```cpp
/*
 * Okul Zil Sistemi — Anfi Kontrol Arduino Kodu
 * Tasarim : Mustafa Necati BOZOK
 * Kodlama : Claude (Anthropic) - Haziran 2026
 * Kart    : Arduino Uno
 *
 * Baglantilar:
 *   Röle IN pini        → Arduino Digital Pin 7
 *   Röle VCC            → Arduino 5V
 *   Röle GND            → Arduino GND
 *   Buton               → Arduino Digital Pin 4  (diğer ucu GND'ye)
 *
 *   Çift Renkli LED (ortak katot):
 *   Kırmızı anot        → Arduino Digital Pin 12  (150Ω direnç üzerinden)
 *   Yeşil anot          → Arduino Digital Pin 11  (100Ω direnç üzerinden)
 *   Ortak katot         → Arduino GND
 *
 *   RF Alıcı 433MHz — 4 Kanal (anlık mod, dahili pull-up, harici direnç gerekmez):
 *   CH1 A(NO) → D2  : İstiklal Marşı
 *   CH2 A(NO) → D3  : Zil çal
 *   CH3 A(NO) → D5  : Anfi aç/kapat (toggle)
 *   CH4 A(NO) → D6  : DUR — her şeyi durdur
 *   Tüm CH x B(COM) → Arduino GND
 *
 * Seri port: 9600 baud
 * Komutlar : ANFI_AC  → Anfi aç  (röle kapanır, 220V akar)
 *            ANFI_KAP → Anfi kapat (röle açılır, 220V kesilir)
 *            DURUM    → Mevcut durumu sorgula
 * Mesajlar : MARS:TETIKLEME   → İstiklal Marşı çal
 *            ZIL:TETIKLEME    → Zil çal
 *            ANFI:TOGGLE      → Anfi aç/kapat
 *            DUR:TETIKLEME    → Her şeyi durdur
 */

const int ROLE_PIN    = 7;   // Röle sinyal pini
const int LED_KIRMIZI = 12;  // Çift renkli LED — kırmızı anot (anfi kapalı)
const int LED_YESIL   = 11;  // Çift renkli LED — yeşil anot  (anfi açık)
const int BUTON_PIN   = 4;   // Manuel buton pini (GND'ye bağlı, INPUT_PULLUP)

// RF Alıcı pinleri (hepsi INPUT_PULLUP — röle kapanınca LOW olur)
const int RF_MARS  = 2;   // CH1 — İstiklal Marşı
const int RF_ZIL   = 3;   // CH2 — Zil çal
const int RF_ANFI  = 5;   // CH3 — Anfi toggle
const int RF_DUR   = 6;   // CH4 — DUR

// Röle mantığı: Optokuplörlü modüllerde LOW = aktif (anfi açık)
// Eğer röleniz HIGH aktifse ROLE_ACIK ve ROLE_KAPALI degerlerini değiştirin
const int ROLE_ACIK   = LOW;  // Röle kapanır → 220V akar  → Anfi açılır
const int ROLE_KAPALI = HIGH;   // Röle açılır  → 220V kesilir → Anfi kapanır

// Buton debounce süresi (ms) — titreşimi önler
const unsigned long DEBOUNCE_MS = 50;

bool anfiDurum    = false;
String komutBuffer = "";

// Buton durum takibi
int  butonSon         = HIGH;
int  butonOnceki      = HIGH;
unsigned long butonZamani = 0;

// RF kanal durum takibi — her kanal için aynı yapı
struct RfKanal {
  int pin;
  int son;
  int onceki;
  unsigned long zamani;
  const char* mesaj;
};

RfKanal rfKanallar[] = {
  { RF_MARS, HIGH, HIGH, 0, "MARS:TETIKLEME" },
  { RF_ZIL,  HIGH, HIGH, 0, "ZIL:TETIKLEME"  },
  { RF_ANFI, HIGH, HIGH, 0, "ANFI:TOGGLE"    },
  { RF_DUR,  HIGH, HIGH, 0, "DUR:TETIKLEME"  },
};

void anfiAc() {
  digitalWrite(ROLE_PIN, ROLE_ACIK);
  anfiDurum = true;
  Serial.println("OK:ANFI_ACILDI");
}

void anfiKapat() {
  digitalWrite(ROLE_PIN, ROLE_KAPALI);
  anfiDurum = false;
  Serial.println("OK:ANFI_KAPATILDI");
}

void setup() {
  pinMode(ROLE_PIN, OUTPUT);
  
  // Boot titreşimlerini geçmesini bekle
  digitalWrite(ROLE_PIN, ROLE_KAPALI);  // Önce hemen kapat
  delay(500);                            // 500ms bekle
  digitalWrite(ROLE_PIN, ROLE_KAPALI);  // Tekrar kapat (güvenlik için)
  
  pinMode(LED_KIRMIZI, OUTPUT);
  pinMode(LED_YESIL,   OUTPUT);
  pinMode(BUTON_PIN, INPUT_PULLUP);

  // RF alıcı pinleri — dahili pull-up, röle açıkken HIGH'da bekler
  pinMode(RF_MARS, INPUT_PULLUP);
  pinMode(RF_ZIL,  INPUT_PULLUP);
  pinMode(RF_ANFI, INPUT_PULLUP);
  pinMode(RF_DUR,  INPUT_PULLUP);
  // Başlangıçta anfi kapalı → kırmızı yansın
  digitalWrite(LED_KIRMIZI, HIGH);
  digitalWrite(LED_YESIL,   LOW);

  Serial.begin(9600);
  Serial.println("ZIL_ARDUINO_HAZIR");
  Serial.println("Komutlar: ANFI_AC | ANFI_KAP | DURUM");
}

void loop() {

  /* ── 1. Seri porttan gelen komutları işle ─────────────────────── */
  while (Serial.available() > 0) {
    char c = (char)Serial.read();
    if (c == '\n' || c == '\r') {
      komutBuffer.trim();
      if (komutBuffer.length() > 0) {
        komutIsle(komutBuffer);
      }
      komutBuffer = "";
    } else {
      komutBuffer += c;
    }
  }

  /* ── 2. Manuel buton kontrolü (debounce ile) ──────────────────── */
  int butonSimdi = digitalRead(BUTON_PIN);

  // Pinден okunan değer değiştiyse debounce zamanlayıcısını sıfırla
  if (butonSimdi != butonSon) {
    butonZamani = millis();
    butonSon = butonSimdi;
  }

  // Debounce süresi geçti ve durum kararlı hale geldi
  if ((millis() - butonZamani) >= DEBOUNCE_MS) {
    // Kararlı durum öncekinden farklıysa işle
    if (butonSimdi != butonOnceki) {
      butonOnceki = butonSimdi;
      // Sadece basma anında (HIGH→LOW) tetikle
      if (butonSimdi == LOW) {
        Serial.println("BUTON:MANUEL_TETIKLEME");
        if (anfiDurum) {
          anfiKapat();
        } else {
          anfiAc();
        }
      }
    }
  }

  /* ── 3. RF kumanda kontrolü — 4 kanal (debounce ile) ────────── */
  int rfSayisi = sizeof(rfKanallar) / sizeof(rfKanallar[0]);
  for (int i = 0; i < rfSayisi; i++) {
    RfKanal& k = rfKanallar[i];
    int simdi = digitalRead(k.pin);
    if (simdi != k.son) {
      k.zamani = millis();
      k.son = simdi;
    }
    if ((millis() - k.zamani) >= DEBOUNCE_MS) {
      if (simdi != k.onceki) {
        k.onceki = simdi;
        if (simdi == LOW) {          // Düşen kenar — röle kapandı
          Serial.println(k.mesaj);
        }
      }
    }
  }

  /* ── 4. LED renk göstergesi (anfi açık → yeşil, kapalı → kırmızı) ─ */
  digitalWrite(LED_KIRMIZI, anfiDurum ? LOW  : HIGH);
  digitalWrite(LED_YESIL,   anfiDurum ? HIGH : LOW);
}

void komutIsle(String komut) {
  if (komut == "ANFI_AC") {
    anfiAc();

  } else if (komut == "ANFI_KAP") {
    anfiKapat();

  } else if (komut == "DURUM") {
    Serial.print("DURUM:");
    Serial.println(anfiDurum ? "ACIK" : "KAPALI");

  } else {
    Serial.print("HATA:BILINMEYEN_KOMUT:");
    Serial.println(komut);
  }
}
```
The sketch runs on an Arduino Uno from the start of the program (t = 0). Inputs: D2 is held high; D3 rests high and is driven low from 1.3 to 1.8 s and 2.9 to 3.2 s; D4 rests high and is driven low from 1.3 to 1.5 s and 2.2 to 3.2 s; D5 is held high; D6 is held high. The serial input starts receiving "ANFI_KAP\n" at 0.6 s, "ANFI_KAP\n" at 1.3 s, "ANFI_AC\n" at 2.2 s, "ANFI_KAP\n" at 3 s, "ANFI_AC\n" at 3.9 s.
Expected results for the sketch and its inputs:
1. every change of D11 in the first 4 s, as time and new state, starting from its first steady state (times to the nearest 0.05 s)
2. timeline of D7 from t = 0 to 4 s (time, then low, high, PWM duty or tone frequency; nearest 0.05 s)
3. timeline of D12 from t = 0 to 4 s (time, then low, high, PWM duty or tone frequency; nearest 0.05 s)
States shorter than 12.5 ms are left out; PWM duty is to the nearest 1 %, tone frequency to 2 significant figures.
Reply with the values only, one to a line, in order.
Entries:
0.5 s low; 1.35 s high; 2.25 s low; 3.9 s high
0 s high; 1.35 s low; 2.25 s high; 3.9 s low
0.5 s high; 1.35 s low; 2.25 s high; 3.9 s low
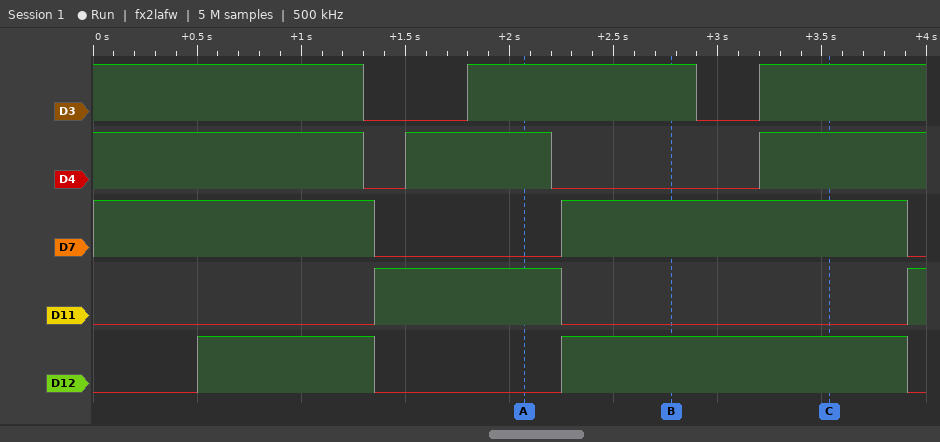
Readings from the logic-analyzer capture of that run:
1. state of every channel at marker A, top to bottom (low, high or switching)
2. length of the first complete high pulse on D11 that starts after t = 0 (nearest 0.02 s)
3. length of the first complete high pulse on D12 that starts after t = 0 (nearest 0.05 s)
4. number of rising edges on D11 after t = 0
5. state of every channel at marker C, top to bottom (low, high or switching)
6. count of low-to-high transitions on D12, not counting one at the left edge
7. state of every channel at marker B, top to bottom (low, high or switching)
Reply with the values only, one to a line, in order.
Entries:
D3 high, D4 high, D7 low, D11 high, D12 low
0.90 s
0.85 s
2
D3 high, D4 high, D7 high, D11 low, D12 high
2
D3 high, D4 low, D7 high, D11 low, D12 high
